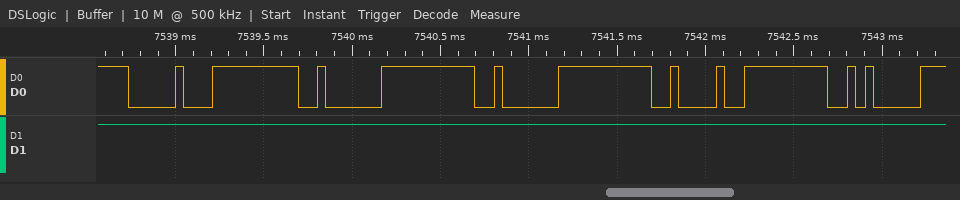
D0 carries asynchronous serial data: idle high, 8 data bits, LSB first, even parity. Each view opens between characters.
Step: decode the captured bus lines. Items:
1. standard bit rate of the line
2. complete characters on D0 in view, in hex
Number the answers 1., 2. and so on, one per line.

1. 19200 baud
2. 10, 02, 02, 42, 0A
